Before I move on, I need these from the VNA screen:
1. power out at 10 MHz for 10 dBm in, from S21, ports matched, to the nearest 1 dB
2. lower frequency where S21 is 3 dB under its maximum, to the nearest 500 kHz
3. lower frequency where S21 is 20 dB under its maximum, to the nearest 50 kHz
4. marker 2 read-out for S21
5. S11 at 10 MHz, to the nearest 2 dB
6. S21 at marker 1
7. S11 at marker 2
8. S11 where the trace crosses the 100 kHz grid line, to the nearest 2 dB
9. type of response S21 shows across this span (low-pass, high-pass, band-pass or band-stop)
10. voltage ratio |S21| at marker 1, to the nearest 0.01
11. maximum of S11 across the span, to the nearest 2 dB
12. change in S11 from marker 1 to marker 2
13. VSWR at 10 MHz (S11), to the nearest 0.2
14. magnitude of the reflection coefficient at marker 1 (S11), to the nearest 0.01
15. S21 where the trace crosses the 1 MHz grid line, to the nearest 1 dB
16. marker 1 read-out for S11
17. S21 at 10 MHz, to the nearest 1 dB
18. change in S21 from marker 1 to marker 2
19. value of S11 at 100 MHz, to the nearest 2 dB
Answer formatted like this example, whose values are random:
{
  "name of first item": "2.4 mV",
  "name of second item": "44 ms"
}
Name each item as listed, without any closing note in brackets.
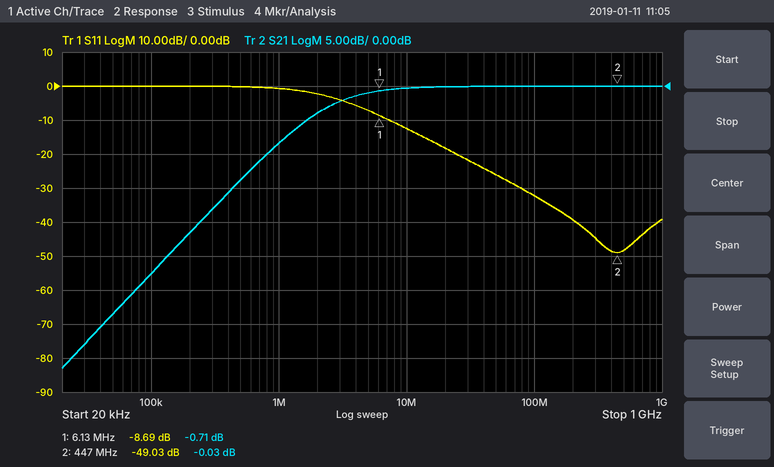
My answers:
{
  "power out at 10 MHz for 10 dBm in, from S21, ports matched, to the nearest 1 dB": "10 dBm",
  "lower frequency where S21 is 3 dB under its maximum, to the nearest 500 kHz": "2.5 MHz",
  "lower frequency where S21 is 20 dB under its maximum, to the nearest 50 kHz": "250 kHz",
  "marker 2 read-out for S21": "-0.03 dB",
  "S11 at 10 MHz, to the nearest 2 dB": "-12 dB",
  "S21 at marker 1": "-0.71 dB",
  "S11 at marker 2": "-49.03 dB",
  "S11 where the trace crosses the 100 kHz grid line, to the nearest 2 dB": "0 dB",
  "type of response S21 shows across this span": "high-pass",
  "voltage ratio |S21| at marker 1, to the nearest 0.01": "0.92",
  "maximum of S11 across the span, to the nearest 2 dB": "0 dB",
  "change in S11 from marker 1 to marker 2": "-40.34 dB",
  "VSWR at 10 MHz (S11), to the nearest 0.2": "1.6",
  "magnitude of the reflection coefficient at marker 1 (S11), to the nearest 0.01": "0.37",
  "S21 where the trace crosses the 1 MHz grid line, to the nearest 1 dB": "-8 dB",
  "marker 1 read-out for S11": "-8.69 dB",
  "S21 at 10 MHz, to the nearest 1 dB": "0 dB",
  "change in S21 from marker 1 to marker 2": "0.68 dB",
  "value of S11 at 100 MHz, to the nearest 2 dB": "-32 dB"
}
